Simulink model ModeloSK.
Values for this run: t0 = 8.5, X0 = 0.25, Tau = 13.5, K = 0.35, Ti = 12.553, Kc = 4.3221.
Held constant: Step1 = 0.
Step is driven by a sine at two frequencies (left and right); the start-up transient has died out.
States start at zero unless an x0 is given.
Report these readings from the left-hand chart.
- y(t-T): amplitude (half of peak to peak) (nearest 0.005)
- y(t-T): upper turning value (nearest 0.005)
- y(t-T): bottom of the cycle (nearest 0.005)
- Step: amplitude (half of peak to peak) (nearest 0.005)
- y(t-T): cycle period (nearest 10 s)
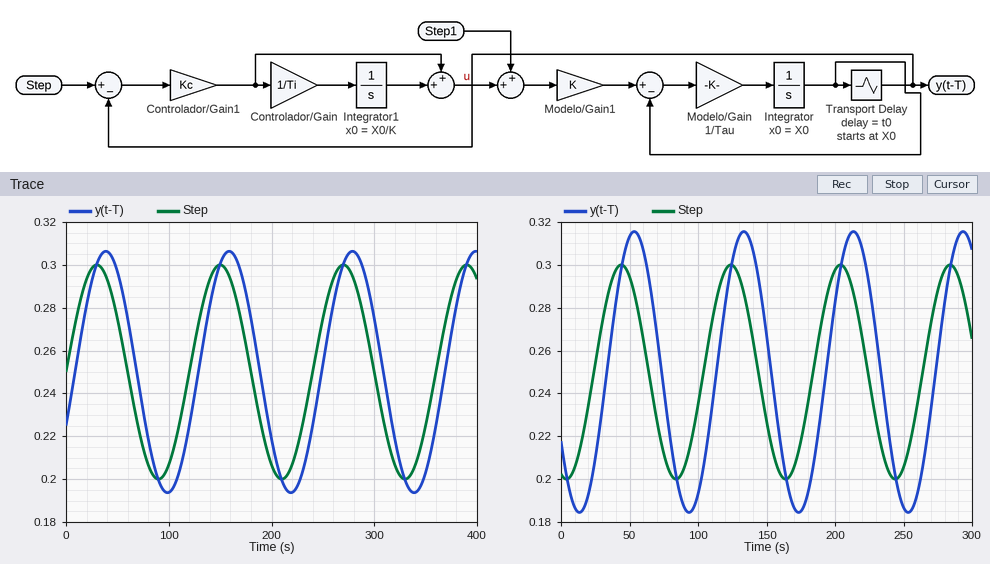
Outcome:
0.055
0.305
0.195
0.050
120 s
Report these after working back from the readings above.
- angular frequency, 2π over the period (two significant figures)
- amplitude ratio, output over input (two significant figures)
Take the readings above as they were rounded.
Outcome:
0.052 rad/s
1.1
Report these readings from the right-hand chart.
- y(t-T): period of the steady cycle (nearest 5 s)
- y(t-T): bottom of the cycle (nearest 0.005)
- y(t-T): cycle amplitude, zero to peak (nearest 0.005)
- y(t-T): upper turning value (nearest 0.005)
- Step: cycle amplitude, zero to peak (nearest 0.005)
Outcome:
80 s
0.185
0.065
0.315
0.050
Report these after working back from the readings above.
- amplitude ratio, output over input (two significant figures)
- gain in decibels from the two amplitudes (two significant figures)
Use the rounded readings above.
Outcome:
1.3
2.3 dB
